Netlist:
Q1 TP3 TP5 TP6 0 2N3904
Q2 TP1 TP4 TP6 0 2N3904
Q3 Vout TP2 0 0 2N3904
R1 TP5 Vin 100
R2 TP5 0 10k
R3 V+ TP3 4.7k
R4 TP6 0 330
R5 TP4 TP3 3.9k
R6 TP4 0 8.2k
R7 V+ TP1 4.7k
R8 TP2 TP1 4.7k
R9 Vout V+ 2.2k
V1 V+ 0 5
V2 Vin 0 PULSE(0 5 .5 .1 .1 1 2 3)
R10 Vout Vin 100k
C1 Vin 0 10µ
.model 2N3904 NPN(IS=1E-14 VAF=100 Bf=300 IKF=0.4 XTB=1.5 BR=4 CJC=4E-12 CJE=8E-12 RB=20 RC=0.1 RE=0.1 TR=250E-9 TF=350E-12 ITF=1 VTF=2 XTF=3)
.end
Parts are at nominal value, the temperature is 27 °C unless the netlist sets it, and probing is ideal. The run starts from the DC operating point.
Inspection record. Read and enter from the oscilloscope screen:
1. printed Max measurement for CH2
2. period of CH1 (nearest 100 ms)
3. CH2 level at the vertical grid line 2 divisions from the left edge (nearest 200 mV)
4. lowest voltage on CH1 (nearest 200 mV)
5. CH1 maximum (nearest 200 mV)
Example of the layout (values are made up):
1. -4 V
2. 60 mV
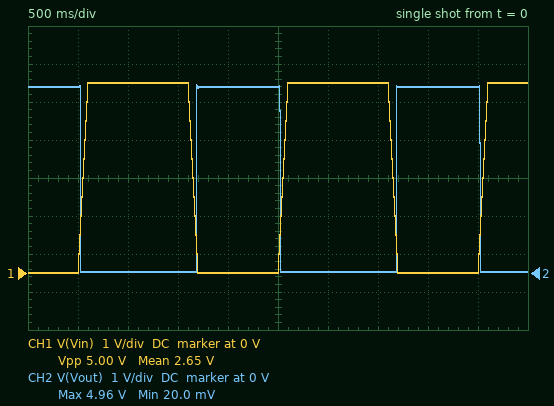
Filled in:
1. 4.96 V
2. 2.0 s
3. 0 V
4. 0 V
5. 5.0 V
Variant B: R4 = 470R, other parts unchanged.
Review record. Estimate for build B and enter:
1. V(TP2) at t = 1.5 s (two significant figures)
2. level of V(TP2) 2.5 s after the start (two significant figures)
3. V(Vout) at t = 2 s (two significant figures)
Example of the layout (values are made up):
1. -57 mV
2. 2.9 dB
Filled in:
1. 700 mV
2. 590 mV
3. 4.7 V
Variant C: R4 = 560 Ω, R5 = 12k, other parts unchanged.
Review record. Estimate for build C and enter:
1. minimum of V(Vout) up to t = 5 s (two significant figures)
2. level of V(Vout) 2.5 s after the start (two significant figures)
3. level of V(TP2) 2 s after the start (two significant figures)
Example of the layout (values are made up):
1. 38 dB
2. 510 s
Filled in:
1. 24 mV
2. 4.6 V
3. 600 mV
